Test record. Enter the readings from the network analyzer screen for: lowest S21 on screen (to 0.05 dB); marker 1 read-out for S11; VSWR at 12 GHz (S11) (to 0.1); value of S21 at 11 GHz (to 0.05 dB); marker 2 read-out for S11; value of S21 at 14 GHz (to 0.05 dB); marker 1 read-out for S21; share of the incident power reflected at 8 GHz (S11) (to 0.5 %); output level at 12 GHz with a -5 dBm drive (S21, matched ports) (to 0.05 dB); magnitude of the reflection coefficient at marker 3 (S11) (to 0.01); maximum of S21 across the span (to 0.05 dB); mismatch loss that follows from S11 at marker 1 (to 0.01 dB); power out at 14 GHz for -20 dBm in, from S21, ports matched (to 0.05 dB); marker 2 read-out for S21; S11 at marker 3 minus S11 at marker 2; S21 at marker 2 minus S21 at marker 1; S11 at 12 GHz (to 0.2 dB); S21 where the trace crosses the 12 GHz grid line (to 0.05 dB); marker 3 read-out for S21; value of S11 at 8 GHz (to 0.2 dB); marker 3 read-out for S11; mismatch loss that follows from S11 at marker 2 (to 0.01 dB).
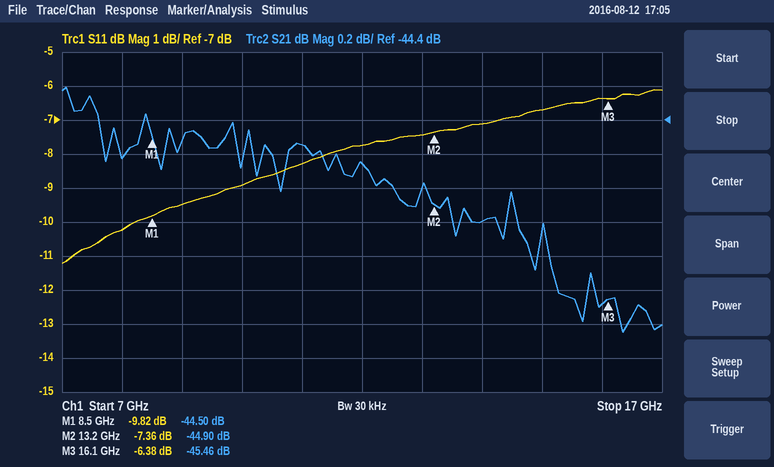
-45.65 dB
-9.82 dB
2.4
-44.55 dB
-7.36 dB
-45.00 dB
-44.50 dB
9.5 %
-49.65 dBm
0.48
-44.20 dB
0.48 dB
-65.00 dBm
-44.90 dB
0.98 dB
-0.40 dB
-7.8 dB
-44.65 dB
-45.46 dB
-10.2 dB
-6.38 dB
0.88 dB
